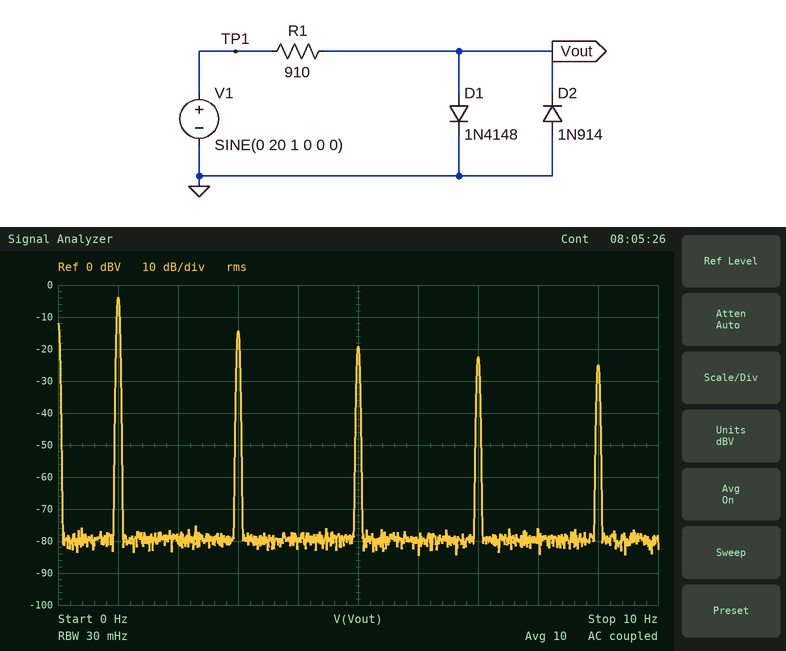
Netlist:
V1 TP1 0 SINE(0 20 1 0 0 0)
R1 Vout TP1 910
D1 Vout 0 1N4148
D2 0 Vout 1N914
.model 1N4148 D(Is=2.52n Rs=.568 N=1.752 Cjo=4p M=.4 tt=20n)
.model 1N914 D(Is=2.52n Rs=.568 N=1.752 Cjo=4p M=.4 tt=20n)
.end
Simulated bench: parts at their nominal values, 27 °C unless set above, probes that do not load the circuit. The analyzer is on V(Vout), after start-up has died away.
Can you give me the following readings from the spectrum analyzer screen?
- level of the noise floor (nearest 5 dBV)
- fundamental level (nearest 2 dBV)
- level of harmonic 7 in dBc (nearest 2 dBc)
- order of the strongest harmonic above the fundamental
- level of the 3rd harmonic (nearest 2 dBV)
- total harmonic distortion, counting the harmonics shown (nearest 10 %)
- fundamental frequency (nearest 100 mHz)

-80 dBV
-4 dBV
-18 dBc
3
-14 dBV
40 %
1.0 Hz
